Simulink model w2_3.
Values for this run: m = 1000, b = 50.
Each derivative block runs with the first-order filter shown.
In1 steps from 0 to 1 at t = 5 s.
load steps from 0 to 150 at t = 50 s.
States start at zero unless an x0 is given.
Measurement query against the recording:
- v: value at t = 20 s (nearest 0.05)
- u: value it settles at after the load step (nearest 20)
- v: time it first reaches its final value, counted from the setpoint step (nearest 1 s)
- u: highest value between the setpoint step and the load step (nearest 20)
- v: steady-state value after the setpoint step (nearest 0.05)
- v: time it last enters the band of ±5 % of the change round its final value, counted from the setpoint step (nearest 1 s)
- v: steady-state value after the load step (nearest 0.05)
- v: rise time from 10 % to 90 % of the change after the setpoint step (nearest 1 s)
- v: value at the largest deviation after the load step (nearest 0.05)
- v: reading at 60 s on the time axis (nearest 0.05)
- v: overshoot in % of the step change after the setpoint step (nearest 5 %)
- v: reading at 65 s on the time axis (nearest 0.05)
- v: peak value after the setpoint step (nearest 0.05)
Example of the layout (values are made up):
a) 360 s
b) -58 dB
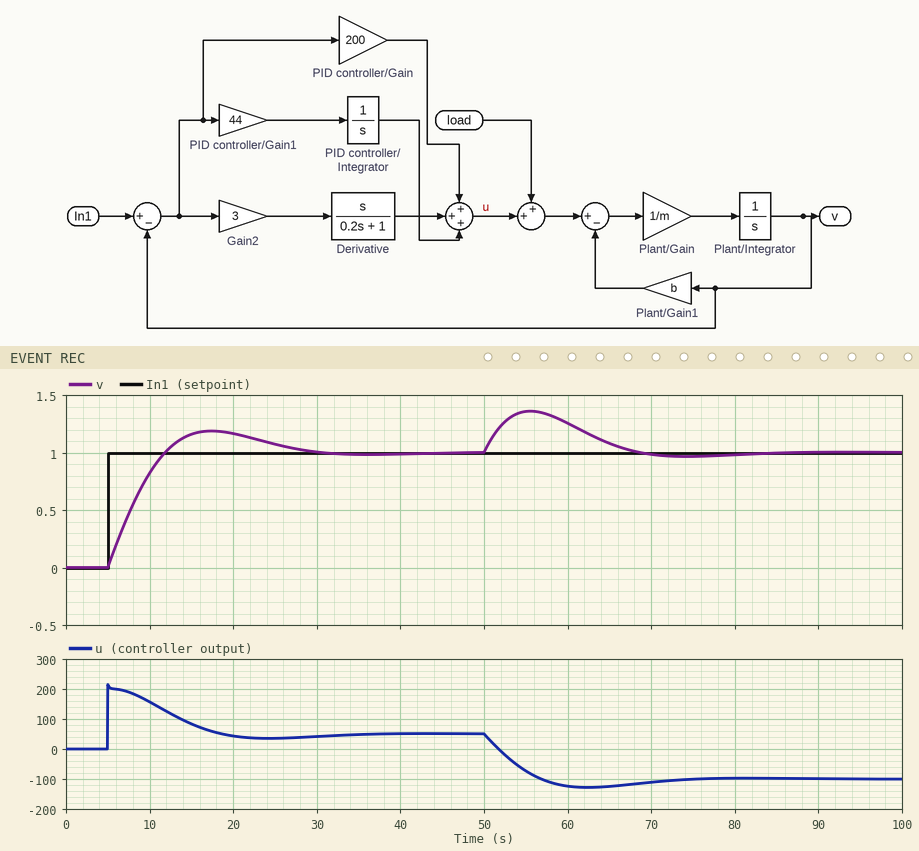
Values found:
a) 1.15
b) -100
c) 7 s
d) 220
e) 1.00
f) 21 s
g) 1.00
h) 5 s
i) 1.35
j) 1.25
k) 20 %
l) 1.10
m) 1.20
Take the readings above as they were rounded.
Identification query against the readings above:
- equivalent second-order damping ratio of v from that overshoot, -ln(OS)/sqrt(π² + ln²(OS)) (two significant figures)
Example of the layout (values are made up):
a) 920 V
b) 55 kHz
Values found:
a) 0.46
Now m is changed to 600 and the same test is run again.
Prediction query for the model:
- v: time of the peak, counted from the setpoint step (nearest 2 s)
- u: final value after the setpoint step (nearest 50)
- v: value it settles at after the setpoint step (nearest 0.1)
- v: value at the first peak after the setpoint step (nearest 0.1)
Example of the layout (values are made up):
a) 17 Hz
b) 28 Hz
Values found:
a) 10 s
b) 50
c) 1.0
d) 1.1
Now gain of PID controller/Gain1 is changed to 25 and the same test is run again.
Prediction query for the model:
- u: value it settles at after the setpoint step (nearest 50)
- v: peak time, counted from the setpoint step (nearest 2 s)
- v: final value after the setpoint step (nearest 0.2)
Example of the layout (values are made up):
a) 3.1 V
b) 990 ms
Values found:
a) 50
b) 16 s
c) 1.0
